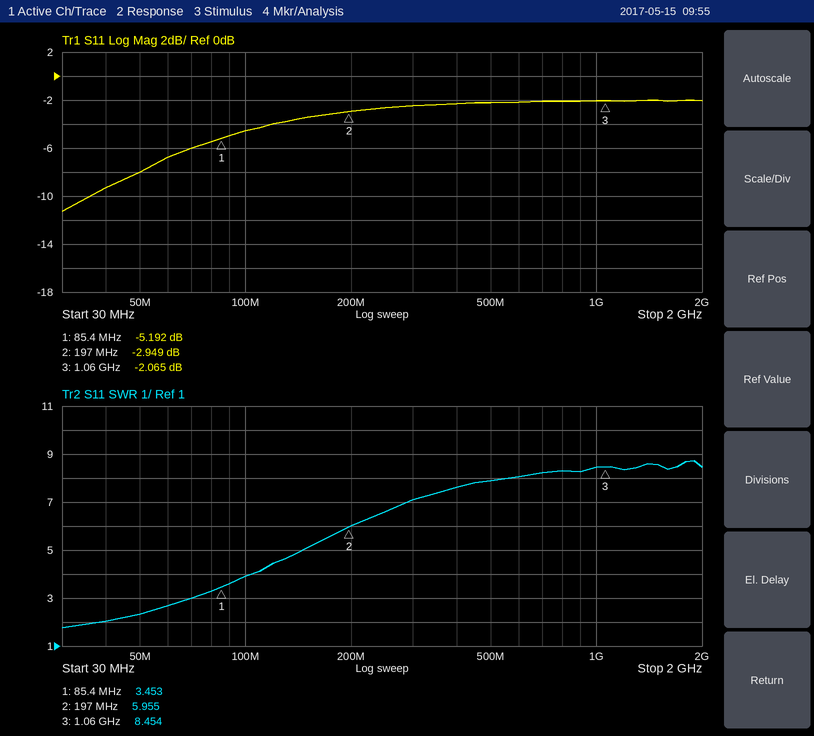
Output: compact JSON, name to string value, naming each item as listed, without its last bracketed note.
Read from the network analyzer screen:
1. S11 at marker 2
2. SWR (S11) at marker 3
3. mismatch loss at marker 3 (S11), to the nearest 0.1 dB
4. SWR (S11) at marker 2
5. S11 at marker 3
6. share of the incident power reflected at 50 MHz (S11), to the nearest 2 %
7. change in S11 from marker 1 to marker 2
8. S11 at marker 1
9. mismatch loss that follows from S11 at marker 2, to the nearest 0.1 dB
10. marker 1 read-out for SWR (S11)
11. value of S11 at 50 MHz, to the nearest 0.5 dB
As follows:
{"S11 at marker 2": "-2.949 dB", "SWR (S11) at marker 3": "8.454", "mismatch loss at marker 3 (S11), to the nearest 0.1 dB": "4.2 dB", "SWR (S11) at marker 2": "5.955", "S11 at marker 3": "-2.065 dB", "share of the incident power reflected at 50 MHz (S11), to the nearest 2 %": "16 %", "change in S11 from marker 1 to marker 2": "2.243 dB", "S11 at marker 1": "-5.192 dB", "mismatch loss that follows from S11 at marker 2, to the nearest 0.1 dB": "3.1 dB", "marker 1 read-out for SWR": "3.453", "value of S11 at 50 MHz, to the nearest 0.5 dB": "-8.0 dB"}
